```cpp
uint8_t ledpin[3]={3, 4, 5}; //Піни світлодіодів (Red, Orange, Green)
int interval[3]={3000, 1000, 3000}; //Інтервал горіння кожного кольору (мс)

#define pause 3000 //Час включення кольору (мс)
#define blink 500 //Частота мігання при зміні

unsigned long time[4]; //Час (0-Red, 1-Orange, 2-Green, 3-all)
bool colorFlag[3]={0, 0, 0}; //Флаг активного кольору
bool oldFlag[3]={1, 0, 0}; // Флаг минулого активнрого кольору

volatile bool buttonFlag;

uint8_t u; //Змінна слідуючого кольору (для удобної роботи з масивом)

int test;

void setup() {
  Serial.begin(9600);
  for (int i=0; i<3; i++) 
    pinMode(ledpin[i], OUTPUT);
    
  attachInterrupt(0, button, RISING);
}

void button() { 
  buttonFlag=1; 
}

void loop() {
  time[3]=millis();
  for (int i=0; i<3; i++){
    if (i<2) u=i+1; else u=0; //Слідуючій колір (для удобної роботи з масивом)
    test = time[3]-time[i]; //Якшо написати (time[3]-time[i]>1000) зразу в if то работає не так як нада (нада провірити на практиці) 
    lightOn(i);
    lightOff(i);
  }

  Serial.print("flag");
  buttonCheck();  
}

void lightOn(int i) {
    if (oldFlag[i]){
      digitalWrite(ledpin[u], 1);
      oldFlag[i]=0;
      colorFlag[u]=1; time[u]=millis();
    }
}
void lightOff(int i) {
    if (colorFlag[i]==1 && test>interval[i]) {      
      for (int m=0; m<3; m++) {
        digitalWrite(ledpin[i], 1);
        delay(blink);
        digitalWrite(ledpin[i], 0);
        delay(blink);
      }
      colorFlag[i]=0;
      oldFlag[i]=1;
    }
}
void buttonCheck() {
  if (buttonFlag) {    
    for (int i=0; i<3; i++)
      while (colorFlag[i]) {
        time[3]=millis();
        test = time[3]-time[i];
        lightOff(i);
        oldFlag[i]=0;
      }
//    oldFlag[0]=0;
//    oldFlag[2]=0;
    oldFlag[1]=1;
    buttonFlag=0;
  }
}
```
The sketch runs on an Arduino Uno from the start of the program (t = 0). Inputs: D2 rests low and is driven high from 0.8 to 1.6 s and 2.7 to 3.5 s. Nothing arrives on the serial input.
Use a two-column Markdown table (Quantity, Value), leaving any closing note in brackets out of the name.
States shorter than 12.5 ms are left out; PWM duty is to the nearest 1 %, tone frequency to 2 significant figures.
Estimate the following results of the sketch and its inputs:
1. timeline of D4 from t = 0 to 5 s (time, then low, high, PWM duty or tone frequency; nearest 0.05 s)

| Quantity | Value |
|---|---|
| timeline of D4 from t = 0 to 5 s | 0 s high; 1.5 s low; 2 s high; 2.5 s low; 3 s high; 3.5 s low |
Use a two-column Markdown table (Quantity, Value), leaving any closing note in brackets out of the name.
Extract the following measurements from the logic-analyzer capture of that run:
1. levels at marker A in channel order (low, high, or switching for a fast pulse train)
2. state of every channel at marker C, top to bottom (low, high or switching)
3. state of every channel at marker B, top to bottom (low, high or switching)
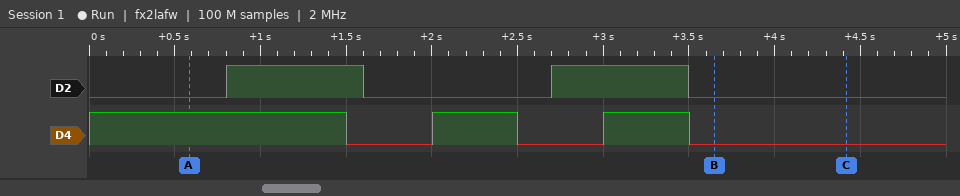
| Quantity | Value |
|---|---|
| levels at marker A in channel order | D2 low, D4 high |
| state of every channel at marker C, top to bottom | D2 low, D4 low |
| state of every channel at marker B, top to bottom | D2 low, D4 low |
